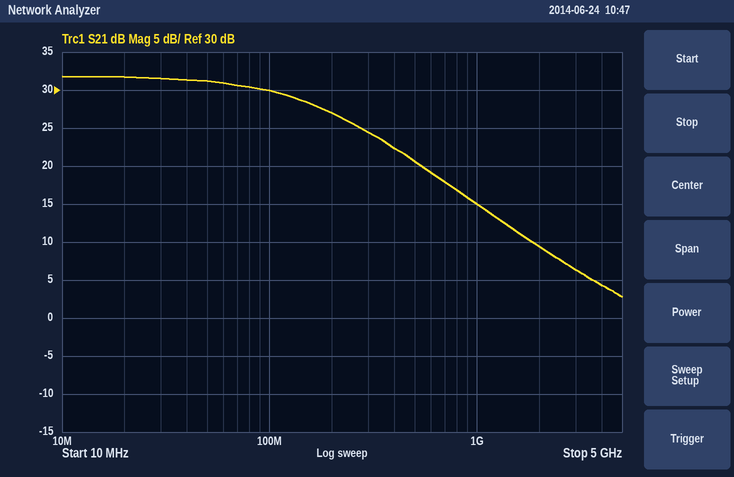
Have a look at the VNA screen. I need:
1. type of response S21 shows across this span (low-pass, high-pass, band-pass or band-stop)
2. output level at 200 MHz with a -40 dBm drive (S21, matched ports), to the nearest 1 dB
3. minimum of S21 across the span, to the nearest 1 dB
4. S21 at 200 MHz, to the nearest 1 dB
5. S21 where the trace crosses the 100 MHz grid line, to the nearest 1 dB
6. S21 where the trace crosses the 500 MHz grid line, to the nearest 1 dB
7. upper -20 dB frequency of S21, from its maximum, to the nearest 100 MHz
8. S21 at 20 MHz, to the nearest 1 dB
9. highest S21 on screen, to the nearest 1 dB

low-pass
-13 dBm
3 dB
27 dB
30 dB
21 dB
1.5 GHz
32 dB
32 dB
